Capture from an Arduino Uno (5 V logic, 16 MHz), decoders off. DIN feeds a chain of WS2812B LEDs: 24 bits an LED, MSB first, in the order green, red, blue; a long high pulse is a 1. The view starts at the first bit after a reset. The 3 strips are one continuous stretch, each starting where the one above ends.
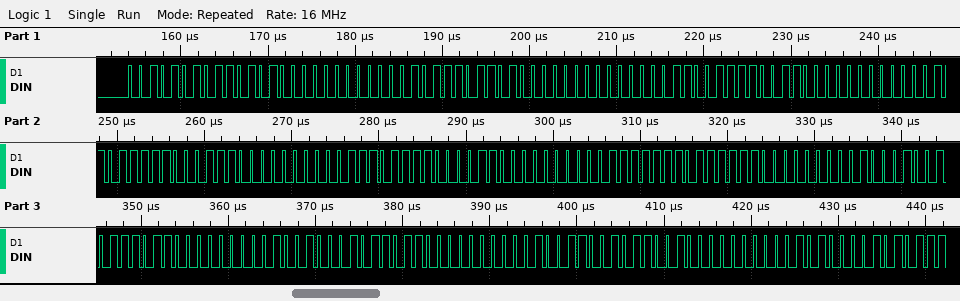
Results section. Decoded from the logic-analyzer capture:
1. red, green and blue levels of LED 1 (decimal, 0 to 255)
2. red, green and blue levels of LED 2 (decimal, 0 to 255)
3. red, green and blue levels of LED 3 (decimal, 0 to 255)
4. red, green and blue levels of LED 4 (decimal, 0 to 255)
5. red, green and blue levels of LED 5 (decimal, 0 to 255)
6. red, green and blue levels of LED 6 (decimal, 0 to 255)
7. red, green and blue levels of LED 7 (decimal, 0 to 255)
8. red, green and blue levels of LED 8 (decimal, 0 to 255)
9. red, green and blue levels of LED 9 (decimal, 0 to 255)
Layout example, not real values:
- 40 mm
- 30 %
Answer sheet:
- 212, 42, 0
- 208, 46, 0
- 204, 51, 0
- 199, 55, 0
- 195, 59, 0
- 191, 63, 0
- 187, 68, 0
- 182, 72, 0
- 178, 76, 0
